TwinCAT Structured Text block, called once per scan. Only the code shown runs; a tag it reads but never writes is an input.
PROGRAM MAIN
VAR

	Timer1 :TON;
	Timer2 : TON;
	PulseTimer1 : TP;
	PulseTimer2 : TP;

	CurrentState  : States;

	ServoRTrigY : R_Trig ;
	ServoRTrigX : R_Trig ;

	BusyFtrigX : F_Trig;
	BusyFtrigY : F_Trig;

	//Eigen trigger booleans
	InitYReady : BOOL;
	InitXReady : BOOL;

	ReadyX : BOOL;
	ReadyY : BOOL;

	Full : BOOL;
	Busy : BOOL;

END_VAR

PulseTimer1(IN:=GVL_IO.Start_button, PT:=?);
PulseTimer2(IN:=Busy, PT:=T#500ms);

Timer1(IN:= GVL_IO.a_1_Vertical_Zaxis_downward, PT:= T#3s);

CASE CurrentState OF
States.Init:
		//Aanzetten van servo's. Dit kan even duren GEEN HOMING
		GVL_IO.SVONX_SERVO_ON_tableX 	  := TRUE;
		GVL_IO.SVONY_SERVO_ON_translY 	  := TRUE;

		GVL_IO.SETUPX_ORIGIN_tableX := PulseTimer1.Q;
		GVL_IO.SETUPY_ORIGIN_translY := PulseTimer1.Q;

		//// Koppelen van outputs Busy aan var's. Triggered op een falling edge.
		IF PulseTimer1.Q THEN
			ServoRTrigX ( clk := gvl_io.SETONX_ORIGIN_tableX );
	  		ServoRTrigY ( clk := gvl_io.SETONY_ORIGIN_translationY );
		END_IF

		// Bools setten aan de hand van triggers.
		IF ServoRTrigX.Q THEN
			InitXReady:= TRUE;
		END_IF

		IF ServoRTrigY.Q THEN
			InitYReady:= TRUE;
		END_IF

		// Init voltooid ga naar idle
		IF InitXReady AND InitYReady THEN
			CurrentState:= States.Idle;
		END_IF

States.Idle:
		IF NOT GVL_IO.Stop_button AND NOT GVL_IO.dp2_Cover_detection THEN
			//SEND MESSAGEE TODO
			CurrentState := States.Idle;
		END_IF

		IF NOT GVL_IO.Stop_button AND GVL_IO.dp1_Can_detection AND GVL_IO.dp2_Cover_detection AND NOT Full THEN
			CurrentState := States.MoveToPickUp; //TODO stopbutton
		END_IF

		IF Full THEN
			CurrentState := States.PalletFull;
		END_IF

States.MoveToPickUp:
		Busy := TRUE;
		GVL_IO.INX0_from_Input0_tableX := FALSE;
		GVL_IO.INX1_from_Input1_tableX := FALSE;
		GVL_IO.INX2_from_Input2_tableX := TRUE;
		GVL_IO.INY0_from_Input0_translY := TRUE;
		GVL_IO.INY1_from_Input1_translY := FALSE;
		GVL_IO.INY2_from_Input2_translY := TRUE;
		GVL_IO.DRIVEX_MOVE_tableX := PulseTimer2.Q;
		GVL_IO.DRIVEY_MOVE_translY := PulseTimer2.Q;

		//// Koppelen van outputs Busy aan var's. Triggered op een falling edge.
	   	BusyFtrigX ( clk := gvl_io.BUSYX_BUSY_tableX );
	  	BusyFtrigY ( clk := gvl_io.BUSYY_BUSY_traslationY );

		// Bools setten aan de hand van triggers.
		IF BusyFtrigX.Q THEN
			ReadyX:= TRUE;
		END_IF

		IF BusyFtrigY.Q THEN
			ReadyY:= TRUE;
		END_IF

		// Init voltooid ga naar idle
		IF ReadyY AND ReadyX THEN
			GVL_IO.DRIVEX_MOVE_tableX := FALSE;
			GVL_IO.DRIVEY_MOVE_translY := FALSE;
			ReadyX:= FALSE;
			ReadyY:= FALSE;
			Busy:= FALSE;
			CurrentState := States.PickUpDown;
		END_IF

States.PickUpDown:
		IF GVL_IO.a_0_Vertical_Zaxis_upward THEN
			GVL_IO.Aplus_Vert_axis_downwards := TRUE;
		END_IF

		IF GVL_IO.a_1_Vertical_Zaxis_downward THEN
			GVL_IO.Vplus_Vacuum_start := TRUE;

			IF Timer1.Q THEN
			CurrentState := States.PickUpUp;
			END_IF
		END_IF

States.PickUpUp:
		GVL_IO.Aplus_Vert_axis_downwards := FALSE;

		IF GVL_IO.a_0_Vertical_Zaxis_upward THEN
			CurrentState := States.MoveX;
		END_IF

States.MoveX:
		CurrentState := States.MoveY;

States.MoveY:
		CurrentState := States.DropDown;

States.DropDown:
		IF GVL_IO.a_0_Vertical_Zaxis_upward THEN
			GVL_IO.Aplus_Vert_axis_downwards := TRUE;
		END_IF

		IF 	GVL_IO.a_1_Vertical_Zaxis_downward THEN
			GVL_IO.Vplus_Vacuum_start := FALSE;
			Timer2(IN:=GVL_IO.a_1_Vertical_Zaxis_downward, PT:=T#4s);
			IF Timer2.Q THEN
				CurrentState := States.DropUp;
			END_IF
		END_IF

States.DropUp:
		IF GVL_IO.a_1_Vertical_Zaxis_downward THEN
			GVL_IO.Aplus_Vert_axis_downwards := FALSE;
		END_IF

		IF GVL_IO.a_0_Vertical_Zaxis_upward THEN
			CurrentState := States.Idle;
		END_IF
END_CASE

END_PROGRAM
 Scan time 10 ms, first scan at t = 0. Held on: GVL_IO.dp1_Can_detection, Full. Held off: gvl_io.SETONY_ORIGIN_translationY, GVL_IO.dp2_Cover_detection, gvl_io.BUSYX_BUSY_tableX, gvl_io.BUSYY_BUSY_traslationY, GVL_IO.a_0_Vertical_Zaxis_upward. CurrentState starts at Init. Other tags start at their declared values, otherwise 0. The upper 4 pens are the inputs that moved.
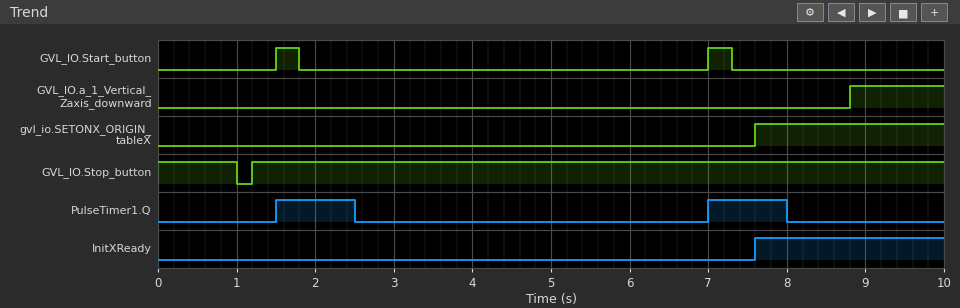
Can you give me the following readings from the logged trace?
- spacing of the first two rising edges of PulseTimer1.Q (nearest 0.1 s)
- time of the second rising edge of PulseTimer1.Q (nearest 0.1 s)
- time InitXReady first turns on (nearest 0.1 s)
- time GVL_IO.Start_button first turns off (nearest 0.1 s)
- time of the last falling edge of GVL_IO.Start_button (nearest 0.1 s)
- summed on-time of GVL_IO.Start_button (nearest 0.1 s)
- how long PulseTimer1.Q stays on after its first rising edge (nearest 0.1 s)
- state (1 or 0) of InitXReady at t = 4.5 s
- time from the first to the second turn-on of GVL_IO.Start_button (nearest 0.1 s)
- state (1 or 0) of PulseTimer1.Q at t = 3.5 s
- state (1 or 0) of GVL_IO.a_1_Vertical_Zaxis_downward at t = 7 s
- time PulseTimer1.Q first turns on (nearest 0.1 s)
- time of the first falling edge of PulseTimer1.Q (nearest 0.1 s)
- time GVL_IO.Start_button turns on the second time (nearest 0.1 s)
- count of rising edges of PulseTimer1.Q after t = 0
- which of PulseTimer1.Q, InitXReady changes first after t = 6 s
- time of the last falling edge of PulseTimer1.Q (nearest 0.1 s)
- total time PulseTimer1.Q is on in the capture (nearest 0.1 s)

5.5 s
7.0 s
7.6 s
1.8 s
7.3 s
0.6 s
1.0 s
0
5.5 s
0
0
1.5 s
2.5 s
7.0 s
2
PulseTimer1.Q
8.0 s
2.0 s
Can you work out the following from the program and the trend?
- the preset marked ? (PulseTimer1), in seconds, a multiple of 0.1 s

1.0 s
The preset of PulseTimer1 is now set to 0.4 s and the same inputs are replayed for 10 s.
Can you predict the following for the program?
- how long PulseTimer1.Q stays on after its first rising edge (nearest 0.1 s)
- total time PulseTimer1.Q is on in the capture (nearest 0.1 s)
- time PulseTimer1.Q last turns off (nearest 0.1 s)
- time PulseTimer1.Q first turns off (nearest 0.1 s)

0.4 s
0.8 s
7.4 s
1.9 s
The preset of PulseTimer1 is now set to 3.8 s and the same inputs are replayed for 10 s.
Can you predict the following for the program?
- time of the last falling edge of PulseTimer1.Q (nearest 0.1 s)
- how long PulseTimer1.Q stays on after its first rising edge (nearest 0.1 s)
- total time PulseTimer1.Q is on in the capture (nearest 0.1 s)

5.3 s
3.8 s
6.8 s
